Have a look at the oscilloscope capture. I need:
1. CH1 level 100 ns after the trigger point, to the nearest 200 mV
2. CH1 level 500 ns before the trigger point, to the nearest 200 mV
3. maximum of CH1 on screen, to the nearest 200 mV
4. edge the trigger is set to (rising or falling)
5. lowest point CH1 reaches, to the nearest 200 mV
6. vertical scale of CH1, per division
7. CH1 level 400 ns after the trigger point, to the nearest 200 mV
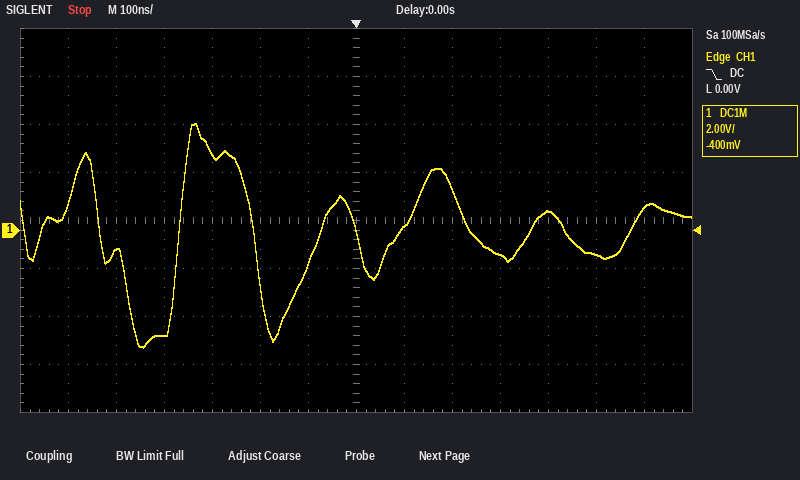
200 mV
-800 mV
4.4 V
falling
-4.8 V
2 V
800 mV
